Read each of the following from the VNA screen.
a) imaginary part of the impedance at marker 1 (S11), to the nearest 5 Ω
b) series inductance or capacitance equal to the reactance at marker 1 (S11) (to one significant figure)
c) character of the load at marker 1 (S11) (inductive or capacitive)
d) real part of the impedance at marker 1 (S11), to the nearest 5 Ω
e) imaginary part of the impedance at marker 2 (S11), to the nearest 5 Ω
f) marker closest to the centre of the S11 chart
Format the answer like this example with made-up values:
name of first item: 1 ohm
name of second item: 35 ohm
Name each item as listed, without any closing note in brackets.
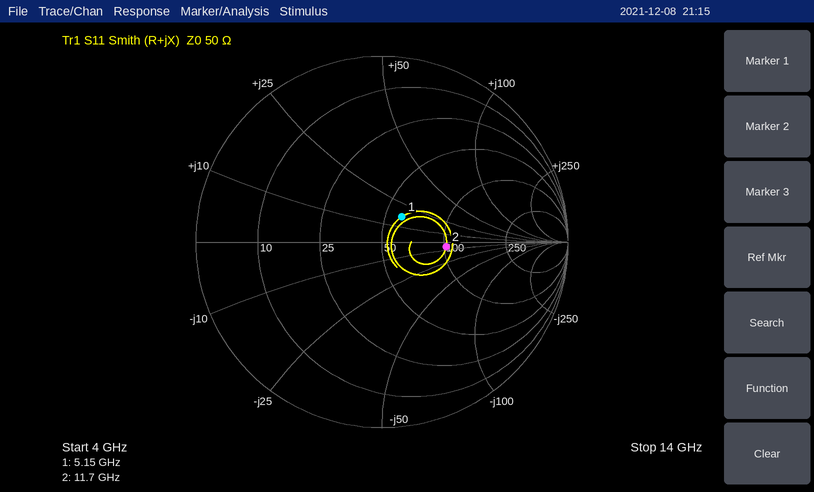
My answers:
imaginary part of the impedance at marker 1 (S11), to the nearest 5 Ω: +15 Ω
series inductance or capacitance equal to the reactance at marker 1 (S11): 500 pH
character of the load at marker 1 (S11): inductive
real part of the impedance at marker 1 (S11), to the nearest 5 Ω: 60 Ω
imaginary part of the impedance at marker 2 (S11), to the nearest 5 Ω: -5 Ω
marker closest to the centre of the S11 chart: marker 1
